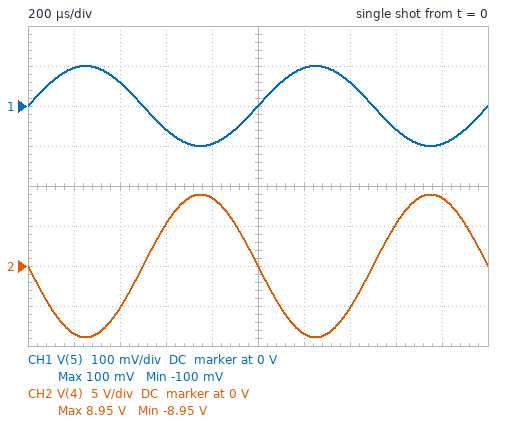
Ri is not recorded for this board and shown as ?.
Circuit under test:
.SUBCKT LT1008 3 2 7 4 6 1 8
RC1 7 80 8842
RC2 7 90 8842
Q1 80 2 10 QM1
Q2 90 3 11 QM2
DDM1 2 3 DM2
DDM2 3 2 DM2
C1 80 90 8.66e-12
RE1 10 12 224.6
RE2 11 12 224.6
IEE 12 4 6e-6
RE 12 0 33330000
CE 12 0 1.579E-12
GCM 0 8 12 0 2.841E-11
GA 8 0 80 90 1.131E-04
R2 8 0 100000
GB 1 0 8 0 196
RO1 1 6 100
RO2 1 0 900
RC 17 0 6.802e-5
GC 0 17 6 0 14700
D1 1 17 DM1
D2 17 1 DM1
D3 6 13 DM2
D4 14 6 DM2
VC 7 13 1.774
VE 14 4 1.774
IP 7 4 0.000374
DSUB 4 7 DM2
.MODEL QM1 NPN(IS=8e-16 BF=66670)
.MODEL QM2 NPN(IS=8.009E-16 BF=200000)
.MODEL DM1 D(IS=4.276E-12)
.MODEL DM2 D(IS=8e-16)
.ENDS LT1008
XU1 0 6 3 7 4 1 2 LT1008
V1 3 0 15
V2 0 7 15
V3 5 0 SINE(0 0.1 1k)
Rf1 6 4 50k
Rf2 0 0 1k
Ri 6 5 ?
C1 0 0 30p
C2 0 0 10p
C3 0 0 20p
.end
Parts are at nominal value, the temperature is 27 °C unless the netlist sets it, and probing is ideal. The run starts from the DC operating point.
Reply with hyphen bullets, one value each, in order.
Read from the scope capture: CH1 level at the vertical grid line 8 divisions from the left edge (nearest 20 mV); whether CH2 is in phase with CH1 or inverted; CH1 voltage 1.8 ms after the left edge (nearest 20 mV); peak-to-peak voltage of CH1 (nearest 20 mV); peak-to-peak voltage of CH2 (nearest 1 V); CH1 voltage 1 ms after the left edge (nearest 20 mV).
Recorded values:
- -60 mV
- inverted
- -100 mV
- 200 mV
- 18 V
- 0 V
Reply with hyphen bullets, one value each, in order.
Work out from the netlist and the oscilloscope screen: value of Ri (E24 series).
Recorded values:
- 560 Ω
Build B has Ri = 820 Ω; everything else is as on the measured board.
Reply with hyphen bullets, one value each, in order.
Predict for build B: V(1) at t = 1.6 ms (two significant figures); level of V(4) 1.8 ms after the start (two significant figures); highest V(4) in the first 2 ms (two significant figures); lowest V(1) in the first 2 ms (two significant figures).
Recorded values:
- 3.6 V
- 5.8 V
- 6.1 V
- -6.1 V
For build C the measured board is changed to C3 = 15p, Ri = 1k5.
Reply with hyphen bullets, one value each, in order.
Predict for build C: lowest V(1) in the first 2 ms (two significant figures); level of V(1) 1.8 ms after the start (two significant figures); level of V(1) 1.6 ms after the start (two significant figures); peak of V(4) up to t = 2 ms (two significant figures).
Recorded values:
- -3.3 V
- 3.2 V
- 2.0 V
- 3.3 V
